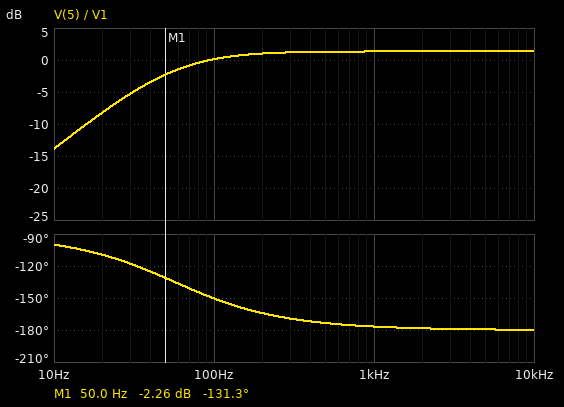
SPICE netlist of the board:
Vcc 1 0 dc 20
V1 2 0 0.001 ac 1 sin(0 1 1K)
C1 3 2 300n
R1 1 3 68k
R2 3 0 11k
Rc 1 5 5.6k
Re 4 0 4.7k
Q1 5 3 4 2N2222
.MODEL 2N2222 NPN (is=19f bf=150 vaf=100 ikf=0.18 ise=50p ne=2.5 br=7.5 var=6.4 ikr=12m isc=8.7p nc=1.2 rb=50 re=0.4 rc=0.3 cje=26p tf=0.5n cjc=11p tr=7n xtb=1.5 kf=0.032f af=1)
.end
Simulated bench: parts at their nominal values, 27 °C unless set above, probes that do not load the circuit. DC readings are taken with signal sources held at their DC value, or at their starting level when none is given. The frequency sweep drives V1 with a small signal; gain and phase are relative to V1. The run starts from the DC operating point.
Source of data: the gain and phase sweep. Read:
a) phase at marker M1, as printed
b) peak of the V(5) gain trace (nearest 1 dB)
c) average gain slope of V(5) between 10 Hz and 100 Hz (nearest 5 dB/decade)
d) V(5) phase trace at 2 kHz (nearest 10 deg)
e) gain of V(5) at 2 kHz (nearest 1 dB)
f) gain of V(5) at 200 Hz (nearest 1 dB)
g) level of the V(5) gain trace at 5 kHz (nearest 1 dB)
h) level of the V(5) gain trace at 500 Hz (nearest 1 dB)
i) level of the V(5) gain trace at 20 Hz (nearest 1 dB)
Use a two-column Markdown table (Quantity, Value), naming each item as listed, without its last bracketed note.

| Quantity | Value |
|---|---|
| phase at marker M1, as printed | -131.3 deg |
| peak of the V(5) gain trace | 1 dB |
| average gain slope of V(5) between 10 Hz and 100 Hz | 15 dB/decade |
| V(5) phase trace at 2 kHz | -180 deg |
| gain of V(5) at 2 kHz | 1 dB |
| gain of V(5) at 200 Hz | 1 dB |
| level of the V(5) gain trace at 5 kHz | 1 dB |
| level of the V(5) gain trace at 500 Hz | 1 dB |
| level of the V(5) gain trace at 20 Hz | -8 dB |
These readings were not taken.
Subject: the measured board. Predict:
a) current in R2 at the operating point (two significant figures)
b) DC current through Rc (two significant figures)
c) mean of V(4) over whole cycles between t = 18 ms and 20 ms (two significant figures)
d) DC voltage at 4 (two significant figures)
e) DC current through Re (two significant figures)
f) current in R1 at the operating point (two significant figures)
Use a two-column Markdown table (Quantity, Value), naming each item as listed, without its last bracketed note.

| Quantity | Value |
|---|---|
| current in R2 at the operating point | 250 µA |
| DC current through Rc | 450 µA |
| mean of V(4) over whole cycles between t = 18 ms and 20 ms | 2.1 V |
| DC voltage at 4 | 2.1 V |
| DC current through Re | 450 µA |
| current in R1 at the operating point | 250 µA |
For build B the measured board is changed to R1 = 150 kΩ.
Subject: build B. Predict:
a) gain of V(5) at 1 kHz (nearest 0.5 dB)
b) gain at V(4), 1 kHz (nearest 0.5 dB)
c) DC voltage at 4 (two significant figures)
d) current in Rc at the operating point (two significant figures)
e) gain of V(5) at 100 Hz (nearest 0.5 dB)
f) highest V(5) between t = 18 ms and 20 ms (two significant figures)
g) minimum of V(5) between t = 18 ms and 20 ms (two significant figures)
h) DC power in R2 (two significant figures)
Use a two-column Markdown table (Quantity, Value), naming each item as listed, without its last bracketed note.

| Quantity | Value |
|---|---|
| gain of V(5) at 1 kHz | 1.0 dB |
| gain at V(4), 1 kHz | -0.5 dB |
| DC voltage at 4 | 760 mV |
| current in Rc at the operating point | 160 µA |
| gain of V(5) at 100 Hz | 0 dB |
| highest V(5) between t = 18 ms and 20 ms | 20 V |
| minimum of V(5) between t = 18 ms and 20 ms | 18 V |
| DC power in R2 | 170 µW |
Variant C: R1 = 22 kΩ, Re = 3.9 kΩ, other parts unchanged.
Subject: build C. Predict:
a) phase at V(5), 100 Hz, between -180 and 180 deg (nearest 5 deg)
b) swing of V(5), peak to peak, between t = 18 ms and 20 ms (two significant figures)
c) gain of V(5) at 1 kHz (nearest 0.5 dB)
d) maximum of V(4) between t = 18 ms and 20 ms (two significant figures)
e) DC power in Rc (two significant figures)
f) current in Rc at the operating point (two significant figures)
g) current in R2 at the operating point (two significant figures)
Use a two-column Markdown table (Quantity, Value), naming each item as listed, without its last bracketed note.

| Quantity | Value |
|---|---|
| phase at V(5), 100 Hz, between -180 and 180 deg | -145 deg |
| swing of V(5), peak to peak, between t = 18 ms and 20 ms | 2.8 V |
| gain of V(5) at 1 kHz | 3.0 dB |
| maximum of V(4) between t = 18 ms and 20 ms | 6.9 V |
| DC power in Rc | 13 mW |
| current in Rc at the operating point | 1.5 mA |
| current in R2 at the operating point | 600 µA |
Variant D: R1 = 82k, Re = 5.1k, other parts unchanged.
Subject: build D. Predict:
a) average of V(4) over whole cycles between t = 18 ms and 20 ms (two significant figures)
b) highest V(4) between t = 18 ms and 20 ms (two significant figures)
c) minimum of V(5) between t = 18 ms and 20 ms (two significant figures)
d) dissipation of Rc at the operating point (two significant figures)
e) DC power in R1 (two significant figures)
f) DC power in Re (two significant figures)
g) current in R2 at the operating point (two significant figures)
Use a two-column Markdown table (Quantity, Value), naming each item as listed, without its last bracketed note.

| Quantity | Value |
|---|---|
| average of V(4) over whole cycles between t = 18 ms and 20 ms | 1.7 V |
| highest V(4) between t = 18 ms and 20 ms | 2.7 V |
| minimum of V(5) between t = 18 ms and 20 ms | 17 V |
| dissipation of Rc at the operating point | 630 µW |
| DC power in R1 | 3.8 mW |
| DC power in Re | 590 µW |
| current in R2 at the operating point | 210 µA |
